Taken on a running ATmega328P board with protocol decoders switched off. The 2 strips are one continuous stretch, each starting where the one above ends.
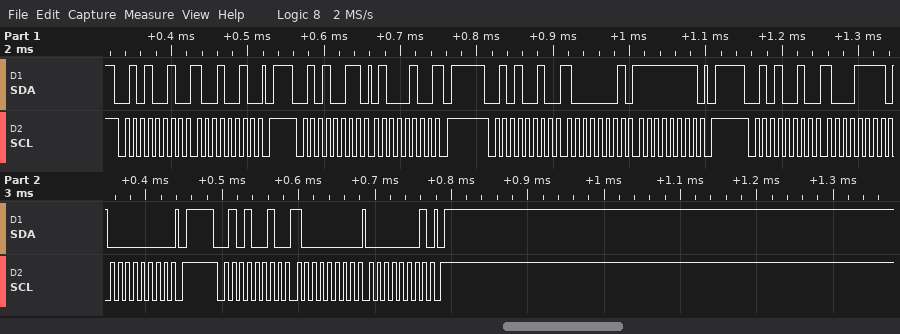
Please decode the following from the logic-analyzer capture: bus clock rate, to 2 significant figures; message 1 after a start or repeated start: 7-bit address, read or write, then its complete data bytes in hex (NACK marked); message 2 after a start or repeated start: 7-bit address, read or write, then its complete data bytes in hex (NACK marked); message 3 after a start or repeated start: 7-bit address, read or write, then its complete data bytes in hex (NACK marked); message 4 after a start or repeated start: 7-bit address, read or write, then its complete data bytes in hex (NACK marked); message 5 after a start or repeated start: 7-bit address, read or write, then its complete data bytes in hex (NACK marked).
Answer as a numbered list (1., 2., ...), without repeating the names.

1. 100 kHz
2. 0x29 write: 92
3. 0x29 read: 44 NACK
4. 0x29 write: 81 FF
5. 0x29 write: 8F 00
6. 0x29 write: 80 01
